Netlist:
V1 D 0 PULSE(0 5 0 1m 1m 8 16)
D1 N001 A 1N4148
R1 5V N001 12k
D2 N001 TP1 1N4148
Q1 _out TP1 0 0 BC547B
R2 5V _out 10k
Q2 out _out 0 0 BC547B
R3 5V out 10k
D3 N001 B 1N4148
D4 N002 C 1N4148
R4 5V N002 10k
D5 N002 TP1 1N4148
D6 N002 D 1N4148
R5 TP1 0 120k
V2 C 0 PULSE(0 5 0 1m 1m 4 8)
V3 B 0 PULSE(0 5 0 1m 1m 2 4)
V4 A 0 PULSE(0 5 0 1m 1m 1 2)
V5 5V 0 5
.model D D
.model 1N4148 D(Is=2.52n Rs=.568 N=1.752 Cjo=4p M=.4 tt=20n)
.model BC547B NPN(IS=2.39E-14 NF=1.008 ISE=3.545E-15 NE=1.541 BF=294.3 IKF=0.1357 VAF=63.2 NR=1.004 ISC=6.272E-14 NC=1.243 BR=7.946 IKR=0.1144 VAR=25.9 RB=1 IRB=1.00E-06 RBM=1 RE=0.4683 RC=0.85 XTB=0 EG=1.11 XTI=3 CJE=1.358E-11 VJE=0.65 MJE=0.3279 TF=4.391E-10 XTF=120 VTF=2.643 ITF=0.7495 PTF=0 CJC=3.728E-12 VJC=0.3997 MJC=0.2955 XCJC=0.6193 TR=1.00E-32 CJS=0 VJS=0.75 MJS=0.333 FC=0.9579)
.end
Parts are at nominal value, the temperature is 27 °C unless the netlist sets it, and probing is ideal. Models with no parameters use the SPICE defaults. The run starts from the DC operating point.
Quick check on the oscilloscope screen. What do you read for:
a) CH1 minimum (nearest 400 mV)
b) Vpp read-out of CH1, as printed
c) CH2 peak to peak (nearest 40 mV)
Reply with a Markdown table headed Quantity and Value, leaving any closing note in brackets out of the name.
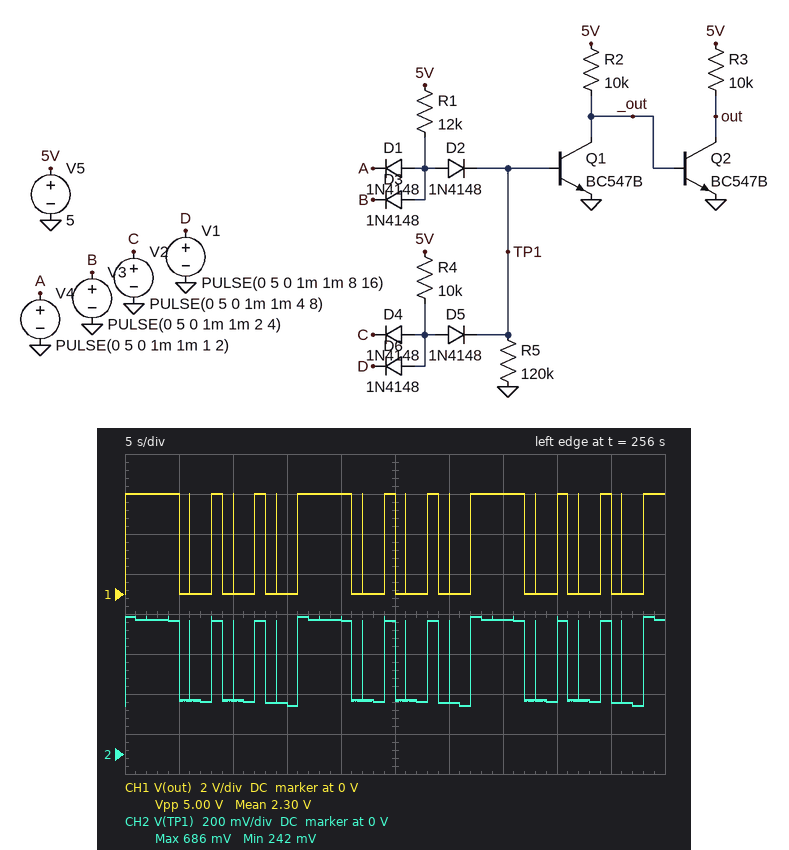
| Quantity | Value |
|---|---|
| CH1 minimum | 0 V |
| Vpp read-out of CH1, as printed | 5.00 V |
| CH2 peak to peak | 440 mV |
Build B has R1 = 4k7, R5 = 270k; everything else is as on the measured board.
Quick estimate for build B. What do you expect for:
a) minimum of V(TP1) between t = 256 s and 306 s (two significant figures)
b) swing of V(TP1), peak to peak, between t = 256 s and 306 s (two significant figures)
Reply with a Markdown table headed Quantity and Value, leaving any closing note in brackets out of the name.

| Quantity | Value |
|---|---|
| minimum of V(TP1) between t = 256 s and 306 s | 290 mV |
| swing of V(TP1), peak to peak, between t = 256 s and 306 s | 410 mV |
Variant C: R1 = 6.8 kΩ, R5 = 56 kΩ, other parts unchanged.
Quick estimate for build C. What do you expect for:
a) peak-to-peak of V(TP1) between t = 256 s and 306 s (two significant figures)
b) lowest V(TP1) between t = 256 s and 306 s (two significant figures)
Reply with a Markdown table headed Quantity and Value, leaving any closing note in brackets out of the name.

| Quantity | Value |
|---|---|
| peak-to-peak of V(TP1) between t = 256 s and 306 s | 470 mV |
| lowest V(TP1) between t = 256 s and 306 s | 220 mV |
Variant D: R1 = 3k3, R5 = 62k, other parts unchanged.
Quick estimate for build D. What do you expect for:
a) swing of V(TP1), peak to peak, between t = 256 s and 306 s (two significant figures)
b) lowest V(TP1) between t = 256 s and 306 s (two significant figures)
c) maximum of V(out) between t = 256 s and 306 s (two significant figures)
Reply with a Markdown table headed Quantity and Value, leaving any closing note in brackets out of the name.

| Quantity | Value |
|---|---|
| swing of V(TP1), peak to peak, between t = 256 s and 306 s | 460 mV |
| lowest V(TP1) between t = 256 s and 306 s | 250 mV |
| maximum of V(out) between t = 256 s and 306 s | 5.0 V |
